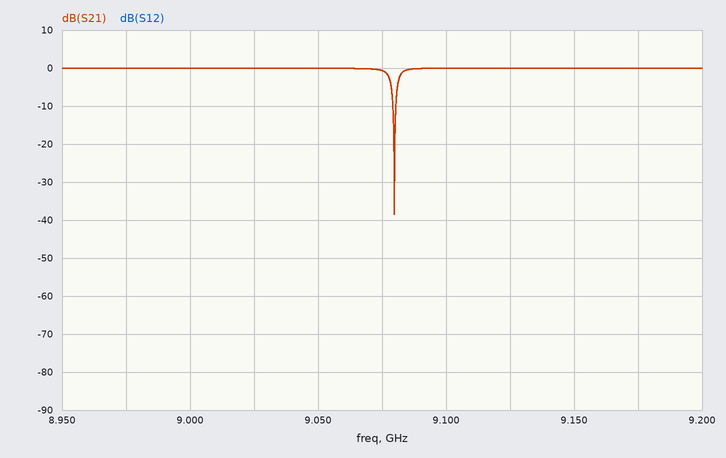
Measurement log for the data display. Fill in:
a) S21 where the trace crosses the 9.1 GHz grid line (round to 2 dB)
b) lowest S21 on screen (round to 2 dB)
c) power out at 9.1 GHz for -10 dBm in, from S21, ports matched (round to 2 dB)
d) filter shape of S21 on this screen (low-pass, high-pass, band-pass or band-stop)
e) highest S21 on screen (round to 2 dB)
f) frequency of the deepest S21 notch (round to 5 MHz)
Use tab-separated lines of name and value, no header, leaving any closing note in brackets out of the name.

S21 where the trace crosses the 9.1 GHz grid line	0 dB
lowest S21 on screen	-38 dB
power out at 9.1 GHz for -10 dBm in, from S21, ports matched	-10 dBm
filter shape of S21 on this screen	band-stop
highest S21 on screen	0 dB
frequency of the deepest S21 notch	9.080 GHz
